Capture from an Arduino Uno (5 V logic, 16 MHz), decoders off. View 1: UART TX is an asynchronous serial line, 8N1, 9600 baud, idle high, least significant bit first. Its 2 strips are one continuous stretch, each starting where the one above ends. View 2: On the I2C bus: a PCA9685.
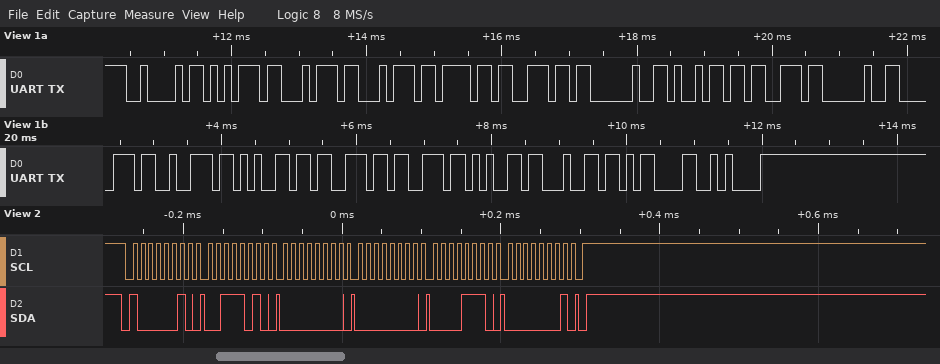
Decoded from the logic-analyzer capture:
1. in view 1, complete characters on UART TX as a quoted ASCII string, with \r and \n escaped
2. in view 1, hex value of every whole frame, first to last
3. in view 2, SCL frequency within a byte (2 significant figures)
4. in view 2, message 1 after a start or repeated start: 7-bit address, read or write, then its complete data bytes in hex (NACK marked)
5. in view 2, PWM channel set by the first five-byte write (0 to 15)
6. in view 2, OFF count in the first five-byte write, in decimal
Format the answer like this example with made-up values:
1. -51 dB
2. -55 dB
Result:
1. "Button is pressed\r\n"
2. 42 75 74 74 6F 6E 20 69 73 20 70 72 65 73 73 65 64 0D 0A
3. 100 kHz
4. 0x41 write: 3A 00 00 0E 01
5. 13
6. 270
